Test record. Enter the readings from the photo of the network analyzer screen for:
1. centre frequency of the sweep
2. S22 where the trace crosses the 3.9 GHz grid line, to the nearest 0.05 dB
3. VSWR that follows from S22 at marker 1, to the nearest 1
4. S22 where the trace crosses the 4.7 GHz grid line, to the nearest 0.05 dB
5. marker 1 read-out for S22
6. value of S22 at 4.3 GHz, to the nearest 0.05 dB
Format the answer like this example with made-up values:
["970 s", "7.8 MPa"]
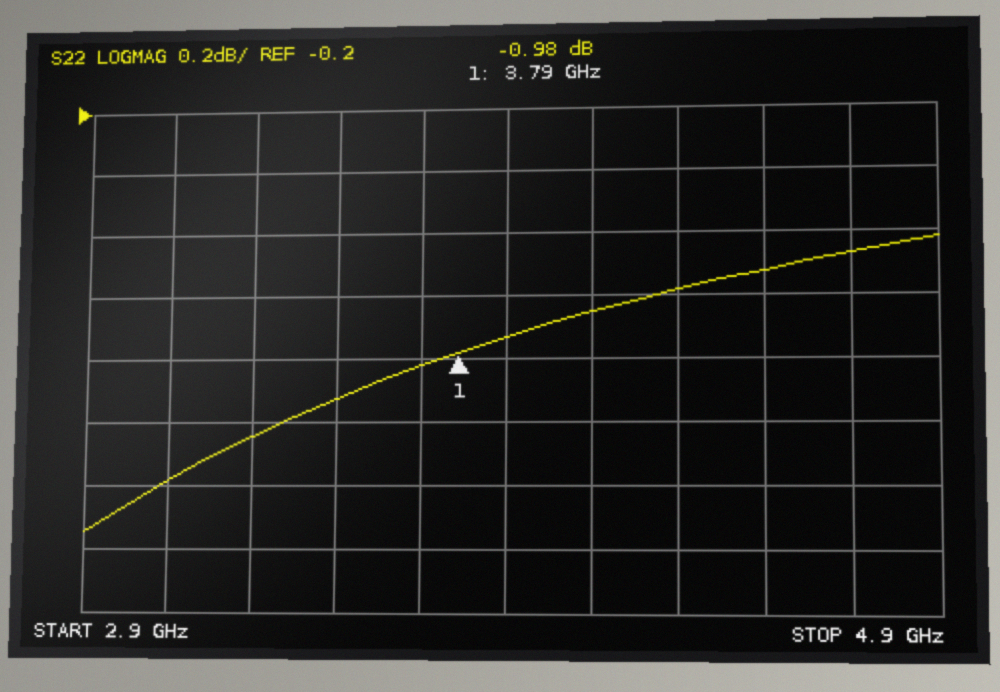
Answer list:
["3.9 GHz", "-0.95 dB", "18", "-0.65 dB", "-0.98 dB", "-0.80 dB"]
